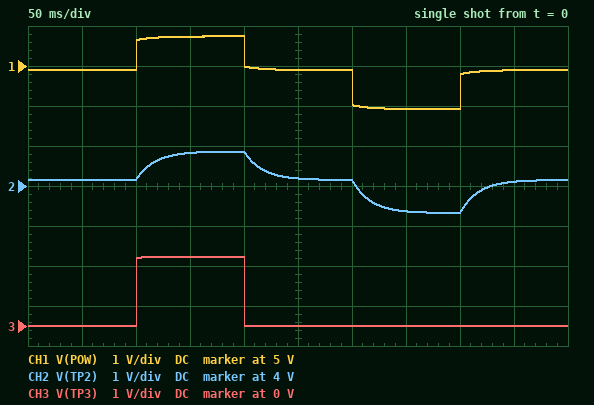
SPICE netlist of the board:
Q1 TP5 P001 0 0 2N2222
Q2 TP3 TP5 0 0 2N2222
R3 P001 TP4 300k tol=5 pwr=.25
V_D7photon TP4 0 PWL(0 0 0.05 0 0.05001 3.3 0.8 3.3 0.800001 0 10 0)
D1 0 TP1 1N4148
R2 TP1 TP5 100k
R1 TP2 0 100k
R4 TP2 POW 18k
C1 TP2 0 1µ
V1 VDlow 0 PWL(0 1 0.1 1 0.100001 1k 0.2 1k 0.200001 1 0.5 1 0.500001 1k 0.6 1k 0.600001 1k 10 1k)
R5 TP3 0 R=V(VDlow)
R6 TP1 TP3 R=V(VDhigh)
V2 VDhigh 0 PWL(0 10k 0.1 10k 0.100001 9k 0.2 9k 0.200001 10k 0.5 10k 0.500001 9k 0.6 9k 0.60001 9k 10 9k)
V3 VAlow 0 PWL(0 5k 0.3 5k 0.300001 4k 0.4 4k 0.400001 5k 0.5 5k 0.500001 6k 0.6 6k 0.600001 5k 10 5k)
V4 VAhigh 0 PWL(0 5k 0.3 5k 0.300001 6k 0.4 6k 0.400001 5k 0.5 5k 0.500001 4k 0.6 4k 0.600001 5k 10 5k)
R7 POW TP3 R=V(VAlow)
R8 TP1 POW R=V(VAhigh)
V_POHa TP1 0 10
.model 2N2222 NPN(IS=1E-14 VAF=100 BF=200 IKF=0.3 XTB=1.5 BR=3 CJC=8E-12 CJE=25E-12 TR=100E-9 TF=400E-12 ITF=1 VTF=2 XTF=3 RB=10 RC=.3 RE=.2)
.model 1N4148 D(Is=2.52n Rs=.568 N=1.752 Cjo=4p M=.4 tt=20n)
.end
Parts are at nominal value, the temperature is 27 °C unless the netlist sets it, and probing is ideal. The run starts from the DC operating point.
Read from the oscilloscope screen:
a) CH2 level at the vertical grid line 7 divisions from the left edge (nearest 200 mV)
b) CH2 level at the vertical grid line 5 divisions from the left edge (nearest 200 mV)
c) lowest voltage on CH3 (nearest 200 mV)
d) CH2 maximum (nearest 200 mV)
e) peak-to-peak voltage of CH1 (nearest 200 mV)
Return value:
3.4 V
4.2 V
0 V
4.8 V
1.8 V
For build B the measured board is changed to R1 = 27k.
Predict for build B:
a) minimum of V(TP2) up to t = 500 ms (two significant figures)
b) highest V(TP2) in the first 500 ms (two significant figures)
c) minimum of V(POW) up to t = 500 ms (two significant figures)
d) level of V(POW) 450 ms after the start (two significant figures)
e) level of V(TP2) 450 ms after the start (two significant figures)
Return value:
2.3 V
3.3 V
3.8 V
4.7 V
2.8 V
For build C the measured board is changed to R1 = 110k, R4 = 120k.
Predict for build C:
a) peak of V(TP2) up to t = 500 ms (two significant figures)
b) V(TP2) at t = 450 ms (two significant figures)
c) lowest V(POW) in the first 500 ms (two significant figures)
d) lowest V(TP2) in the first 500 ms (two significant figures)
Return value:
2.7 V
2.2 V
4.0 V
2.0 V
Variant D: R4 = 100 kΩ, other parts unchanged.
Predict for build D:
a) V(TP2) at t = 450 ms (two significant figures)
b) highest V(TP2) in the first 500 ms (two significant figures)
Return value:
2.3 V
2.8 V
